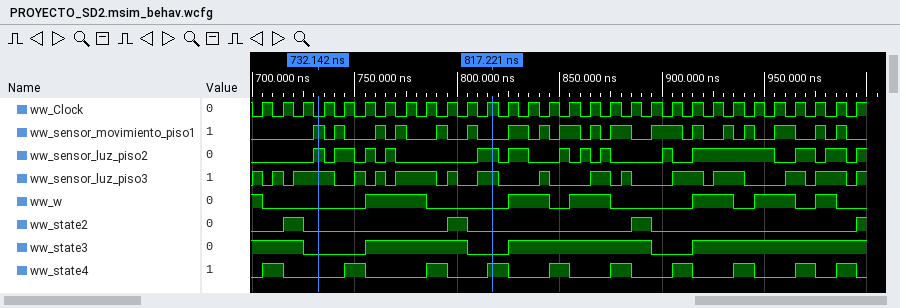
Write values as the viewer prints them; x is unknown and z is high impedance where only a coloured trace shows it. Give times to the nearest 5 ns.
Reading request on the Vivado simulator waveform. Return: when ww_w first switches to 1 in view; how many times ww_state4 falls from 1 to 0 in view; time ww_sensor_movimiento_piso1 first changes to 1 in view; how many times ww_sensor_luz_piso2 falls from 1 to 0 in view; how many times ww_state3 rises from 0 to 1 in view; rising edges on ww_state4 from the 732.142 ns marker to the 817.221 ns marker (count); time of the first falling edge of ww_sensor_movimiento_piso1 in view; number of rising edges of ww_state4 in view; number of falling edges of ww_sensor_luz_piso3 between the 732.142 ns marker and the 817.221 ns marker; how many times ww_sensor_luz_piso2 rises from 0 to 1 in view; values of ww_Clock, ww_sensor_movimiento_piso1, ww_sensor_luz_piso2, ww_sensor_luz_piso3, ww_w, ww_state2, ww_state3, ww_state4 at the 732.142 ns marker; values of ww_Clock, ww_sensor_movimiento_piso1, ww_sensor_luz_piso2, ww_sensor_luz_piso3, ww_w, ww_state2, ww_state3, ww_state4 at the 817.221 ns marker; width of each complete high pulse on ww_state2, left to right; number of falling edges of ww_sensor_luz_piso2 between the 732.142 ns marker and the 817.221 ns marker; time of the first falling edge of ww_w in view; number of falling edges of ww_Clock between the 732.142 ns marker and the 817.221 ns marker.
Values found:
755 ns
10
730 ns
13
3
3
735 ns
10
5
14
ww_Clock=0, ww_sensor_movimiento_piso1=1, ww_sensor_luz_piso2=1, ww_sensor_luz_piso3=1, ww_w=0, ww_state2=0, ww_state3=0, ww_state4=0
ww_Clock=1, ww_sensor_movimiento_piso1=0, ww_sensor_luz_piso2=1, ww_sensor_luz_piso3=1, ww_w=0, ww_state2=0, ww_state3=0, ww_state4=1
10 ns, 10 ns, 10 ns
4
705 ns
8
